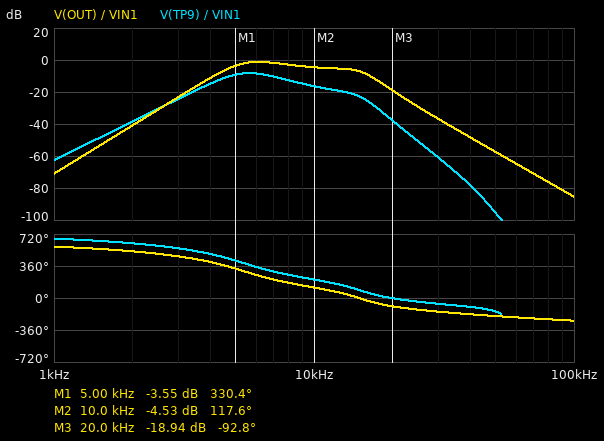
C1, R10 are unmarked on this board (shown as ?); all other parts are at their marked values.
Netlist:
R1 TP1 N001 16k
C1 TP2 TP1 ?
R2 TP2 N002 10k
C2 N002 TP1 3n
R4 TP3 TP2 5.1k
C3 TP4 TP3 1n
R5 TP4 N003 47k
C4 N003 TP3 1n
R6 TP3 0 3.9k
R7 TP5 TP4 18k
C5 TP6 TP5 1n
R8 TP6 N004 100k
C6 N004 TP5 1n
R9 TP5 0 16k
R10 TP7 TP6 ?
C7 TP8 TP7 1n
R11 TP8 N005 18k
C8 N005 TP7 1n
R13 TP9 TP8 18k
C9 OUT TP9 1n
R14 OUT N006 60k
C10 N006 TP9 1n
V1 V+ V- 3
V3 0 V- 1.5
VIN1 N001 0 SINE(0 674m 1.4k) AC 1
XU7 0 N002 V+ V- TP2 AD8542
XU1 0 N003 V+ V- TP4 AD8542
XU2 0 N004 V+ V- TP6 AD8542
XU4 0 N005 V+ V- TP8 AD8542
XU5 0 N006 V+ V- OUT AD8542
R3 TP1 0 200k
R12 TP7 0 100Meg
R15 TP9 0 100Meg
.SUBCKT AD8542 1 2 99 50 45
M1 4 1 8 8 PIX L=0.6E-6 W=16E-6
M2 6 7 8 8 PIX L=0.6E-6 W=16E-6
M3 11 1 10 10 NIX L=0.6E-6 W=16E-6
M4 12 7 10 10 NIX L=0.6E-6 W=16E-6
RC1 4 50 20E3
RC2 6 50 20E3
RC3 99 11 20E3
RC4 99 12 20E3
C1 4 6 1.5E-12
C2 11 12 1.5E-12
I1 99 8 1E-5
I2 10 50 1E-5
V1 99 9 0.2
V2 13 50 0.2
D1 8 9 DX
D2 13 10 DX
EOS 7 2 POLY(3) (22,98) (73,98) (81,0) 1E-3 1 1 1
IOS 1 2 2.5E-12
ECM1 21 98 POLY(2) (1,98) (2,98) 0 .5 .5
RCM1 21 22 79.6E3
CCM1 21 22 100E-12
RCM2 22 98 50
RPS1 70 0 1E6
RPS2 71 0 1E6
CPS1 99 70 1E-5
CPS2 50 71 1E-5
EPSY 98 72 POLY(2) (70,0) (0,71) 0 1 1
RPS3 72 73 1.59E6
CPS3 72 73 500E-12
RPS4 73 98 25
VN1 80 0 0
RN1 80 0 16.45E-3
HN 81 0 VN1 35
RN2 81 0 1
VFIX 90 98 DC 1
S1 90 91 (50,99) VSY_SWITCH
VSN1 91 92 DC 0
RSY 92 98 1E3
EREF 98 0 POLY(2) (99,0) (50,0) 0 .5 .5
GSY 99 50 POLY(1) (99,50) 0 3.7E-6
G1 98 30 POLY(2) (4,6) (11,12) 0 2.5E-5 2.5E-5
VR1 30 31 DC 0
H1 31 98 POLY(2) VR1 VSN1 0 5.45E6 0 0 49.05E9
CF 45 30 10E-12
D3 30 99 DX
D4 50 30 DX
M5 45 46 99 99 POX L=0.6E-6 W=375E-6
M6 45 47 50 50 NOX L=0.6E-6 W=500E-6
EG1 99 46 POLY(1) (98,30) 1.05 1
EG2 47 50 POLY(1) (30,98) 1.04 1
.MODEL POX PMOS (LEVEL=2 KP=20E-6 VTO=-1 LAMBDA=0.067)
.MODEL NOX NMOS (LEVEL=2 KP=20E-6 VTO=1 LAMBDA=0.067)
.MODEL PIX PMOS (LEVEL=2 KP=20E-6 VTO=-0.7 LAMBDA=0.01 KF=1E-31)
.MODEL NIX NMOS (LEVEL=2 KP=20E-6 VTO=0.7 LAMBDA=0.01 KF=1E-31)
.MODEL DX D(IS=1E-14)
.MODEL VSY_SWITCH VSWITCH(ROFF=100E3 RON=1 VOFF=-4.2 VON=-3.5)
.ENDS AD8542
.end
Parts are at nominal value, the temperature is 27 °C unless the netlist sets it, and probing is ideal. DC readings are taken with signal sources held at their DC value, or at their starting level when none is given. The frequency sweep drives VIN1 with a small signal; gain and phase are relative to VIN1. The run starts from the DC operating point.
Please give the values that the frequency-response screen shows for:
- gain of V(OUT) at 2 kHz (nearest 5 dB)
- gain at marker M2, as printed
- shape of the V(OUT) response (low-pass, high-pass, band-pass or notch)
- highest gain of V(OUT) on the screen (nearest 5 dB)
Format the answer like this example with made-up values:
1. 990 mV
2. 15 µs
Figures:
1. -40 dB
2. -4.53 dB
3. band-pass
4. 0 dB
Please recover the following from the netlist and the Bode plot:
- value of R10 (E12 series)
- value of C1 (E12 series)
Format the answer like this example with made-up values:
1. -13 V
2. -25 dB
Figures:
1. 18 kΩ
2. 390 pF
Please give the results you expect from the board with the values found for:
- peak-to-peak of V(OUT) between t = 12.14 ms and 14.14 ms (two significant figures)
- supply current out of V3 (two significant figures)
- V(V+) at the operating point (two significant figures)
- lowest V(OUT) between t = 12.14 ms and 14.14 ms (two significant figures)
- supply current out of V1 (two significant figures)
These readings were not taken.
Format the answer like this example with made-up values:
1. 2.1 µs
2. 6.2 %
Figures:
1. 2.0 mV
2. 140 nA
3. 1.5 V
4. -2.0 mV
5. 240 µA
